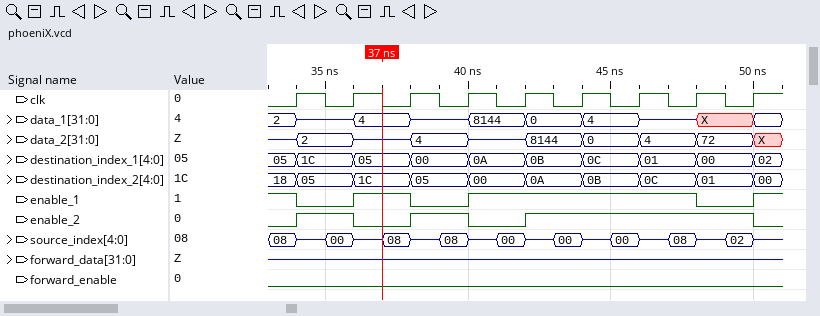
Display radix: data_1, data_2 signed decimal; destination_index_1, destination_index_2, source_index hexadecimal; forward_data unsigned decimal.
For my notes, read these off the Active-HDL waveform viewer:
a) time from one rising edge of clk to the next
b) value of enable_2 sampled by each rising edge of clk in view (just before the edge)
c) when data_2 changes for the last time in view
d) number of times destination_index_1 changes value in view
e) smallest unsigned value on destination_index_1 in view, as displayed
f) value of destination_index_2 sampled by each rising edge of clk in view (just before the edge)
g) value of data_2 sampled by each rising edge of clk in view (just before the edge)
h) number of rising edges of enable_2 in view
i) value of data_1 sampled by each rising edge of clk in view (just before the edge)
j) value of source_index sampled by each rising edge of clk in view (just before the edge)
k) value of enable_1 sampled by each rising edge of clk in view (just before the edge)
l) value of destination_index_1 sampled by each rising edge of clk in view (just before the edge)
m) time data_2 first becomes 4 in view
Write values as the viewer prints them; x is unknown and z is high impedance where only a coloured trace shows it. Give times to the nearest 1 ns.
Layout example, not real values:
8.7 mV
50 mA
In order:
2 ns
0 1 0 1 0 1 1 1 1
50 ns
9
00
18, 05, 1C, 05, 00, 0A, 0B, 0C, 01
z, 2, z, 4, z, 8144, 0, 4, 72
3
2, z, 4, z, 8144, 0, 4, z, X
08, 00, 08, 08, 00, 00, 00, 08, 02
1 0 1 0 1 1 1 1 0
05, 1C, 05, 00, 0A, 0B, 0C, 01, 00
38 ns
